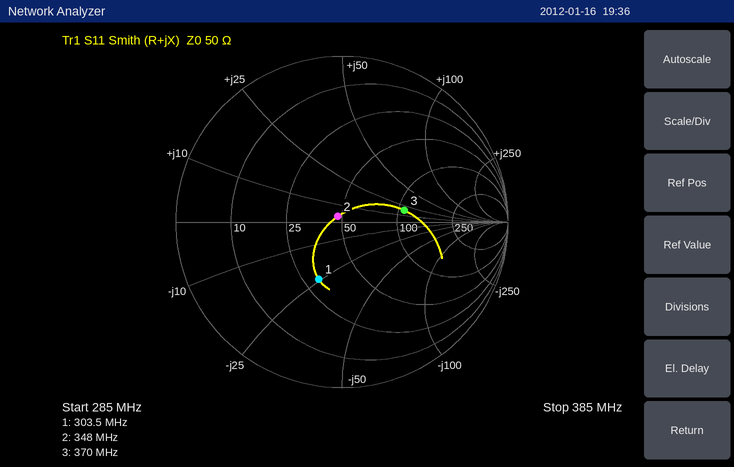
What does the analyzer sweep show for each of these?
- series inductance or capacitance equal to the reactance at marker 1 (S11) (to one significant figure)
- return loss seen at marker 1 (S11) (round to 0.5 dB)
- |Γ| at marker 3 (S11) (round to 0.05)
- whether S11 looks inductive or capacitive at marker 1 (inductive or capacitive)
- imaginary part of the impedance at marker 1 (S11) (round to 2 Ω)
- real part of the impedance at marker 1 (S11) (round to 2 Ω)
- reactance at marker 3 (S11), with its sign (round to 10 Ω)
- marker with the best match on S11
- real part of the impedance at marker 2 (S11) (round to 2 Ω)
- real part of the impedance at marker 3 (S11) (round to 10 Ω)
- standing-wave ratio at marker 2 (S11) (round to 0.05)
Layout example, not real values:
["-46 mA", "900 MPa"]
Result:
["20 pF", "8.5 dB", "0.40", "capacitive", "-24 Ω", "30 Ω", "+20 Ω", "marker 2", "48 Ω", "110 Ω", "1.10"]
